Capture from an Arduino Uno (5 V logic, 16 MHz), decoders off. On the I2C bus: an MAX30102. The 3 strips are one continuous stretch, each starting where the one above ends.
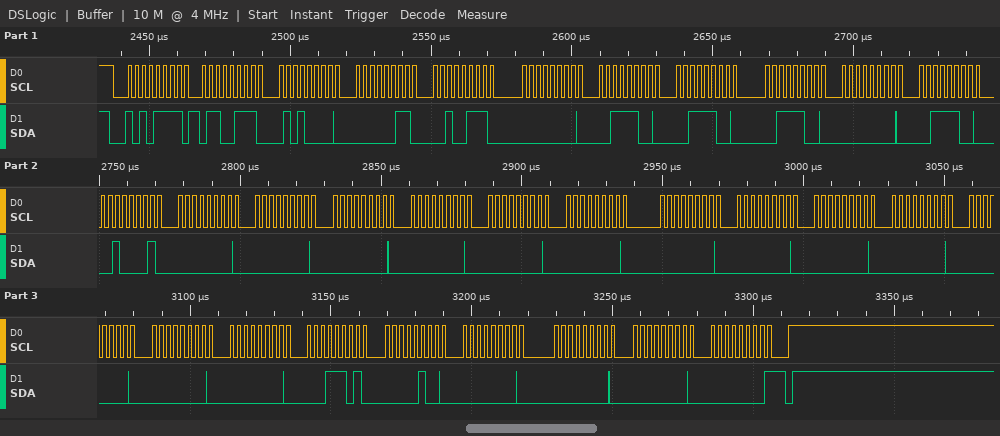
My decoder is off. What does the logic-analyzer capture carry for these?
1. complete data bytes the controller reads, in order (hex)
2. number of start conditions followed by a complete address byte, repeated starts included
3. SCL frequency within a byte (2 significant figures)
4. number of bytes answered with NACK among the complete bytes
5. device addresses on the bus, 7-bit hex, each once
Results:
67 50 03 27 00 3C 3C 3C 00 3C 21 00 00 00 00 00 00 00 00 00 00 00 00 00 1D 04 00 00 00 00
1
400 kHz
1
0x57
